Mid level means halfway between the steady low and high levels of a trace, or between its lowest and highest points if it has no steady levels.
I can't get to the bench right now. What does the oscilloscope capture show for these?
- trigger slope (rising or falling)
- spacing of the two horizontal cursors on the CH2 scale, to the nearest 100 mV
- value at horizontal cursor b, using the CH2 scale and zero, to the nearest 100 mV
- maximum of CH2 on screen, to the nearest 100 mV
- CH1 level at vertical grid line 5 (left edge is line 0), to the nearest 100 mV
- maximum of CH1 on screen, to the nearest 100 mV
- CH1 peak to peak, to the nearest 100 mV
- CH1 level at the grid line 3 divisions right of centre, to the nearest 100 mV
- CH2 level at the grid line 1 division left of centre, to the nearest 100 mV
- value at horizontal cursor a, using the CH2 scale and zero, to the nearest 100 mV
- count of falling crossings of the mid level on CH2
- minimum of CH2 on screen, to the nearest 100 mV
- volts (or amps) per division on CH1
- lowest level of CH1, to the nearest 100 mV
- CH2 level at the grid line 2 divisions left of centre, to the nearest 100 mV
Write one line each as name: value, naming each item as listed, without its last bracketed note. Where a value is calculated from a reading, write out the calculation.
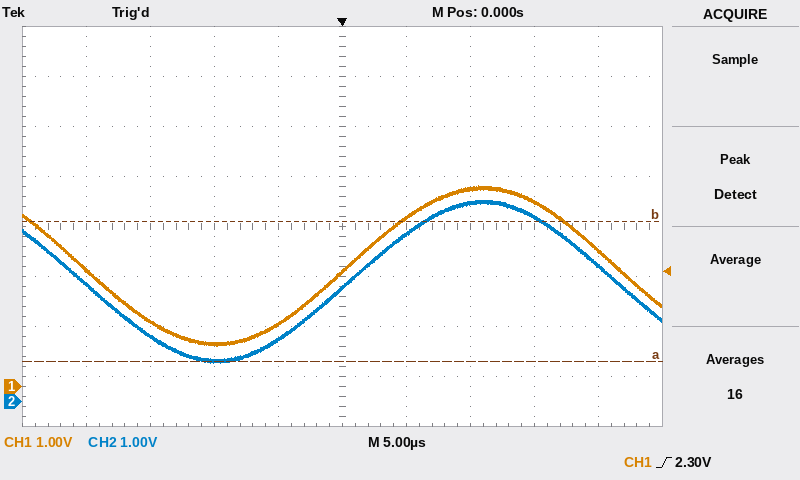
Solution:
trigger slope: rising
spacing of the two horizontal cursors on the CH2 scale, to the nearest 100 mV: 2.8 V
value at horizontal cursor b, using the CH2 scale and zero, to the nearest 100 mV: 3.6 V
maximum of CH2 on screen, to the nearest 100 mV: 4.0 V
CH1 level at vertical grid line 5 (left edge is line 0), to the nearest 100 mV: 2.3 V
maximum of CH1 on screen, to the nearest 100 mV: 4.0 V
CH1 peak to peak, to the nearest 100 mV: 4.0 V − (800 mV) = 3.2 V
CH1 level at the grid line 3 divisions right of centre, to the nearest 100 mV: 3.7 V
CH2 level at the grid line 1 division left of centre, to the nearest 100 mV: 1.2 V
value at horizontal cursor a, using the CH2 scale and zero, to the nearest 100 mV: 800 mV
count of falling crossings of the mid level on CH2: 2
minimum of CH2 on screen, to the nearest 100 mV: 800 mV
volts (or amps) per division on CH1: 1 V
lowest level of CH1, to the nearest 100 mV: 800 mV
CH2 level at the grid line 2 divisions left of centre, to the nearest 100 mV: 800 mV
